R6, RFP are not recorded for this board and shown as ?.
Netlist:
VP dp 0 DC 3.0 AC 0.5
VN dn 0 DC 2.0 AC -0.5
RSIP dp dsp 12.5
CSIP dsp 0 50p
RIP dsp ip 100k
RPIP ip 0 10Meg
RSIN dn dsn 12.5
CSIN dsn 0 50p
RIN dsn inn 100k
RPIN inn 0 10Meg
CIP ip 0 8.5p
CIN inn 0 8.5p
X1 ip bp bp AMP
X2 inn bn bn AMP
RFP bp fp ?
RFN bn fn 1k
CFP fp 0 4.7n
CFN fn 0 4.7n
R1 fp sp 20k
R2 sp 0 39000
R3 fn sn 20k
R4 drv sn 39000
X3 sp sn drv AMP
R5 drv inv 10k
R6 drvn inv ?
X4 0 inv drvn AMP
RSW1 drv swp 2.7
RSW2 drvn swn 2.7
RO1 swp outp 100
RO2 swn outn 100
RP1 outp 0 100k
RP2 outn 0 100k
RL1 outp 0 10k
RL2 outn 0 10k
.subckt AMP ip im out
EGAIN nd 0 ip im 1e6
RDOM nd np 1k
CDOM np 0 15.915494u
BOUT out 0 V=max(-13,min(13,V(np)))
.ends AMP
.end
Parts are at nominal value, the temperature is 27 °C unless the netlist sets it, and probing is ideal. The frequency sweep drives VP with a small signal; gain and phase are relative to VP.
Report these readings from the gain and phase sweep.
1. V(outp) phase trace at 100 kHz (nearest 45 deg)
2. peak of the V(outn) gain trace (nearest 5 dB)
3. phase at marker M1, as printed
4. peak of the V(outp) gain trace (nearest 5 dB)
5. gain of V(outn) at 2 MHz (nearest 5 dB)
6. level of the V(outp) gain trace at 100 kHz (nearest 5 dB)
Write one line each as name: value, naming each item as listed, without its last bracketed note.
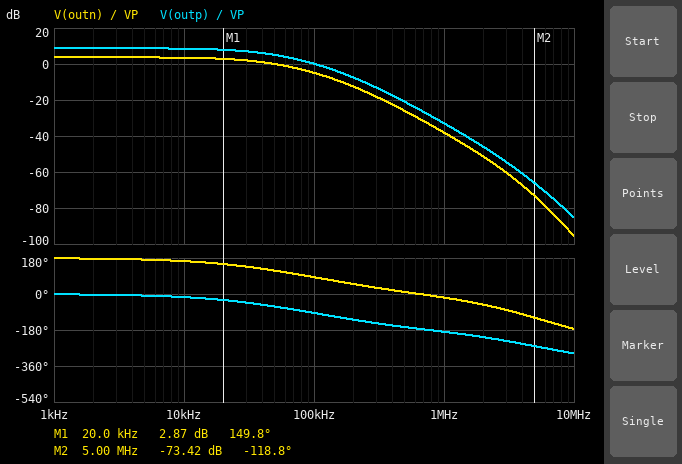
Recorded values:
V(outp) phase trace at 100 kHz: -90 deg
peak of the V(outn) gain trace: 5 dB
phase at marker M1, as printed: 149.8 deg
peak of the V(outp) gain trace: 10 dB
gain of V(outn) at 2 MHz: -50 dB
level of the V(outp) gain trace at 100 kHz: 0 dB
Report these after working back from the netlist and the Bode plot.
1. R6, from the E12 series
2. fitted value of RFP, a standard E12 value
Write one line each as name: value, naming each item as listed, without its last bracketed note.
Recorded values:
R6, from the E12 series: 5.6 kΩ
fitted value of RFP, a standard E12 value: 680 Ω
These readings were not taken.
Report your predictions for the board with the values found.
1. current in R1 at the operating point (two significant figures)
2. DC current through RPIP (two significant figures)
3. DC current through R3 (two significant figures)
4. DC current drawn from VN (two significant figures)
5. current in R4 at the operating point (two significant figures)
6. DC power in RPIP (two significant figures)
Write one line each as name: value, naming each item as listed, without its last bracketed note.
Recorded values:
current in R1 at the operating point: 50 µA
DC current through RPIP: 300 nA
DC current through R3: 1.9 µA
DC current drawn from VN: 200 nA
current in R4 at the operating point: 1.9 µA
DC power in RPIP: 880 nW
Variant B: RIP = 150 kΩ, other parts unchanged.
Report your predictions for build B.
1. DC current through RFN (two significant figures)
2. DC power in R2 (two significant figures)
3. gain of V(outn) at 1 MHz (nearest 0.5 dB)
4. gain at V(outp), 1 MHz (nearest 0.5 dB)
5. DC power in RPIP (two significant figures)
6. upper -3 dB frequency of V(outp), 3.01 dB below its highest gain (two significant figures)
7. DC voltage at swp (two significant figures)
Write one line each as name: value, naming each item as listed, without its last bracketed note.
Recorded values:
DC current through RFN: 2.3 µA
DC power in R2: 96 µW
gain of V(outn) at 1 MHz: -40.5 dB
gain at V(outp), 1 MHz: -35.5 dB
DC power in RPIP: 870 nW
upper -3 dB frequency of V(outp), 3.01 dB below its highest gain: 42 kHz
DC voltage at swp: 1.8 V
